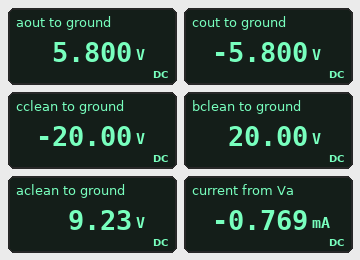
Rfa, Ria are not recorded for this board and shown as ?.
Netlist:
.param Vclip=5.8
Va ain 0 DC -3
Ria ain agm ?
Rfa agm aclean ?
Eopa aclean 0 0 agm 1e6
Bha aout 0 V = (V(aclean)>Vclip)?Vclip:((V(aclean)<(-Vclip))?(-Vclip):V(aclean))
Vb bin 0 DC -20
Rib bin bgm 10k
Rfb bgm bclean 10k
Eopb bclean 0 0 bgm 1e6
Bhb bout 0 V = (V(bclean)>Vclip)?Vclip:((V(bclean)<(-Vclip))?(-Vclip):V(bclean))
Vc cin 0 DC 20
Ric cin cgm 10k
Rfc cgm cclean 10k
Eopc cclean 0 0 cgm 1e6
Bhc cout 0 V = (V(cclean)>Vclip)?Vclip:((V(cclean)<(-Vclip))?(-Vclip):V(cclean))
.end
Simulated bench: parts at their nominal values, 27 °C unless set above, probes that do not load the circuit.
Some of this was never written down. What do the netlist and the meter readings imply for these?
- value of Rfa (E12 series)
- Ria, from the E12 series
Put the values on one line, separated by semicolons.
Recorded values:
12 kΩ; 3.9 kΩ
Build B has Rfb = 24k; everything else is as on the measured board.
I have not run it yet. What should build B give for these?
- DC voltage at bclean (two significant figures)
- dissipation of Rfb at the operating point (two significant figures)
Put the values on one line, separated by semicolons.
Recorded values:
48 V; 96 mW
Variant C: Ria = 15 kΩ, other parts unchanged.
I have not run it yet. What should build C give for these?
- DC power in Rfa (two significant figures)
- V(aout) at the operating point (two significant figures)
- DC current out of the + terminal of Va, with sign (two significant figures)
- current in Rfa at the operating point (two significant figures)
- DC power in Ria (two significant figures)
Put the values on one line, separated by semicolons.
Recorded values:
480 µW; 2.4 V; -200 µA; 200 µA; 600 µW
